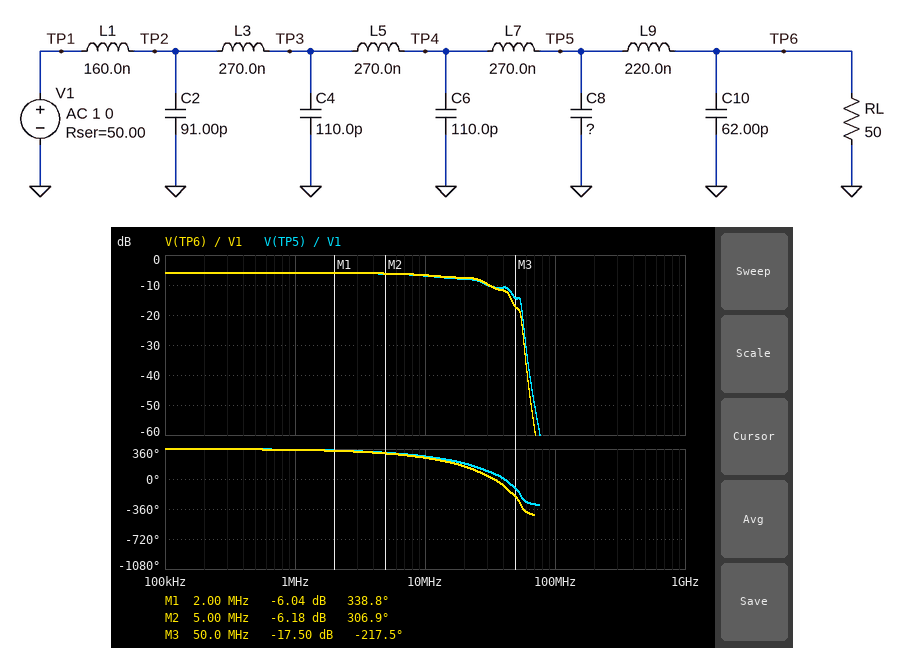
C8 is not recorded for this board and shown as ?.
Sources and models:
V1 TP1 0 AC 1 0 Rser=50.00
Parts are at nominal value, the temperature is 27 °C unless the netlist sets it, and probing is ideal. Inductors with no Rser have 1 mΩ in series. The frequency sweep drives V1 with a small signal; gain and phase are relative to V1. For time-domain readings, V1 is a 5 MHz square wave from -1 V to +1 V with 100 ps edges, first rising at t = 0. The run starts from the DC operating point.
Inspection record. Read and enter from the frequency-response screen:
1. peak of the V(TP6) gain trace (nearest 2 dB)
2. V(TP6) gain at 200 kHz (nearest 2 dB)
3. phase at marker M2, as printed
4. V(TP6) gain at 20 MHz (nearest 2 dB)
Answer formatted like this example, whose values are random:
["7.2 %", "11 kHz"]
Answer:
["-6 dB", "-6 dB", "306.9 deg", "-8 dB"]
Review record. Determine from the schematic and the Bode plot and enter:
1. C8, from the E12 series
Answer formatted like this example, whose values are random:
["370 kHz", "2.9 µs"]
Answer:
["330 pF"]
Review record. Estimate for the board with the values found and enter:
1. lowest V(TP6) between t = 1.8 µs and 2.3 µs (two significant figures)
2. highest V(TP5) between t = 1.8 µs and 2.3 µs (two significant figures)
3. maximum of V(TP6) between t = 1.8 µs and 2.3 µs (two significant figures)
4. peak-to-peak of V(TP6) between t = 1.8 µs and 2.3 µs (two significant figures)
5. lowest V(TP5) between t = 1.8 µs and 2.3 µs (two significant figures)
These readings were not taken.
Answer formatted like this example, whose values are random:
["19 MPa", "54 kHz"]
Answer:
["-540 mV", "520 mV", "540 mV", "1.1 V", "-520 mV"]
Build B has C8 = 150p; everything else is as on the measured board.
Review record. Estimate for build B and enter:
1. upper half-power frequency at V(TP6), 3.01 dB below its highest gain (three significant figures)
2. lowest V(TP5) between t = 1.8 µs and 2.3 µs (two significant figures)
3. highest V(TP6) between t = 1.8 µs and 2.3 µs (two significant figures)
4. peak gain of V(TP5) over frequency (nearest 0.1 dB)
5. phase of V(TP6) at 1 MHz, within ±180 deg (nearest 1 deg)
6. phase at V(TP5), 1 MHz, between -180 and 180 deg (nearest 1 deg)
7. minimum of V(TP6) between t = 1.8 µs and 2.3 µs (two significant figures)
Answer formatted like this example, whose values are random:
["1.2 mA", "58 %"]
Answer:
["55.0 MHz", "-690 mV", "700 mV", "-4.1 dB", "-9 deg", "-7 deg", "-700 mV"]
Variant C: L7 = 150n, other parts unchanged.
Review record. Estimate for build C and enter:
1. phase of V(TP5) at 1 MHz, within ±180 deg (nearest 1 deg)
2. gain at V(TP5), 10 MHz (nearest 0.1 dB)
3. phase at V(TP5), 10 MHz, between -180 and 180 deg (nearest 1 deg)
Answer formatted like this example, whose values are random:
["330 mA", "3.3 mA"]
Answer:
["-9 deg", "-7.1 dB", "-84 deg"]
